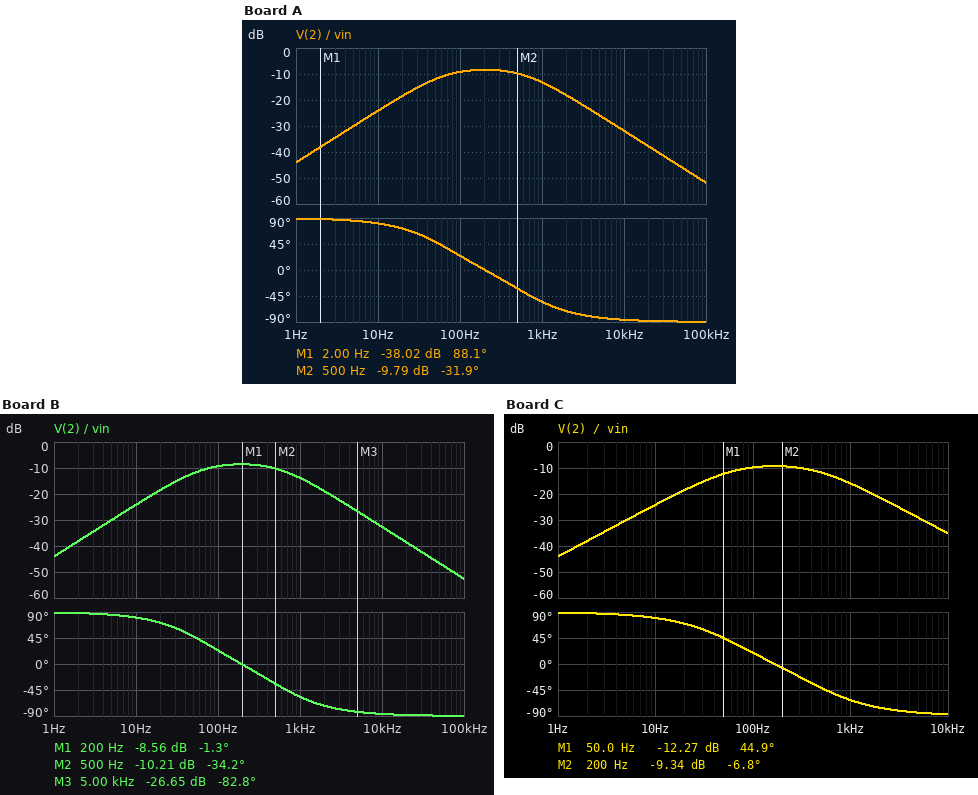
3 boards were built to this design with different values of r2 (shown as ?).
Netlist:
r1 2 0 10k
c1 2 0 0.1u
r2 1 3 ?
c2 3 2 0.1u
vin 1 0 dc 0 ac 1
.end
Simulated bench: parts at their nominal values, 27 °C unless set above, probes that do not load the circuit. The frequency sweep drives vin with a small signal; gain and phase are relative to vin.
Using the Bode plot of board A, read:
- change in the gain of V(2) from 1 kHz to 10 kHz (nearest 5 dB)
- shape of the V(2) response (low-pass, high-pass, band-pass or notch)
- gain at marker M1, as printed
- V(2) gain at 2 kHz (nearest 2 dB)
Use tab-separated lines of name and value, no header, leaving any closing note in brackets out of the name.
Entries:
change in the gain of V(2) from 1 kHz to 10 kHz	-20 dB
shape of the V(2) response	band-pass
gain at marker M1, as printed	-38.02 dB
V(2) gain at 2 kHz	-18 dB
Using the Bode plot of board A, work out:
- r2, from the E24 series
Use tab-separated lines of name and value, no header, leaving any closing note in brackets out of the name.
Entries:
r2, from the E24 series	6.2 kΩ
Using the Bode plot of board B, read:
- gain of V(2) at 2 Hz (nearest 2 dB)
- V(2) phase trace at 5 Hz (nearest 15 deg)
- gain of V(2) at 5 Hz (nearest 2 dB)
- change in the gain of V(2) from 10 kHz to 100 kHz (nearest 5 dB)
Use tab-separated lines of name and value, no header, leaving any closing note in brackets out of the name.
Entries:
gain of V(2) at 2 Hz	-38 dB
V(2) phase trace at 5 Hz	90 deg
gain of V(2) at 5 Hz	-30 dB
change in the gain of V(2) from 10 kHz to 100 kHz	-20 dB
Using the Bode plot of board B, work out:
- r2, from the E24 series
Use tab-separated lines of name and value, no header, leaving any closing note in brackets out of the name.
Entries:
r2, from the E24 series	6.8 kΩ
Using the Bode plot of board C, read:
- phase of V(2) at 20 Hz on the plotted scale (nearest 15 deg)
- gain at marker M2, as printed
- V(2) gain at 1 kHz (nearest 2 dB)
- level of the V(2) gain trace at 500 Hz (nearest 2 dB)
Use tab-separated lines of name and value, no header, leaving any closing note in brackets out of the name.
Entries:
phase of V(2) at 20 Hz on the plotted scale	75 deg
gain at marker M2, as printed	-9.34 dB
V(2) gain at 1 kHz	-16 dB
level of the V(2) gain trace at 500 Hz	-12 dB
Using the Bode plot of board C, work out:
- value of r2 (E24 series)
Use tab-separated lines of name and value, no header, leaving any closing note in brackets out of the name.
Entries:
value of r2	9.1 kΩ
